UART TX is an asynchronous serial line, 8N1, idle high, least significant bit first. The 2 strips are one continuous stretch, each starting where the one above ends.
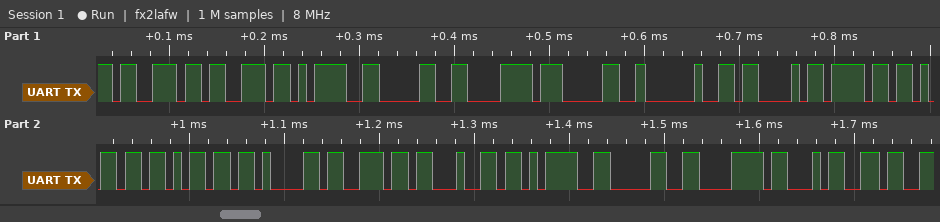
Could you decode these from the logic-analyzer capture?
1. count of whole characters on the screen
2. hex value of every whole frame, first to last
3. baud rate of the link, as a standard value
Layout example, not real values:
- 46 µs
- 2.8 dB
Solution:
- 18
- 73 73 3D 30 78 30 20 43 6F 6D 6D 61 6E 64 3D 30 78 34
- 115200 baud
